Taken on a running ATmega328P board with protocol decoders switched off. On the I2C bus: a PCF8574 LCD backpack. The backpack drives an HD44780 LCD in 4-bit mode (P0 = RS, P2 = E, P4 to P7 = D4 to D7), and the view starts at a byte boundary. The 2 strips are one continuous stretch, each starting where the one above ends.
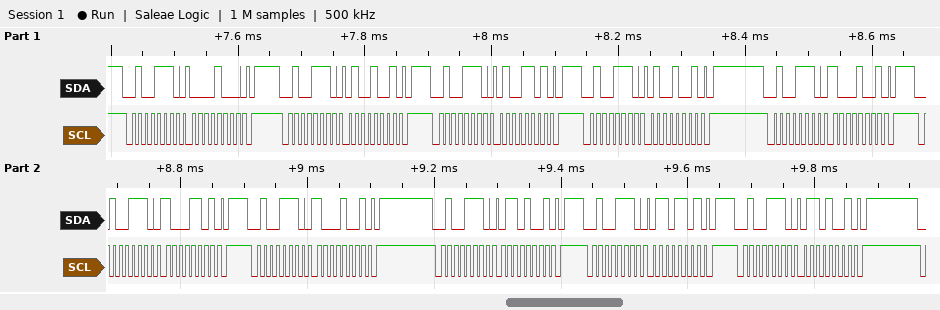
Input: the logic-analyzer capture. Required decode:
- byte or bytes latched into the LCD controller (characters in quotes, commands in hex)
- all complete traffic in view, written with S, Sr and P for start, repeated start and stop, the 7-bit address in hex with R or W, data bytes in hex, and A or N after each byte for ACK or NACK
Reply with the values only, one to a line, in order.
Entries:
'H'
S 27W A 08 A P S 27W A 49 A P S 27W A 4D A P S 27W A 49 A P S 27W A 89 A P S 27W A 8D A P S 27W A 89 A P S 27W A 69 A P S 27W A 6D A P S 27W A 69 A P
